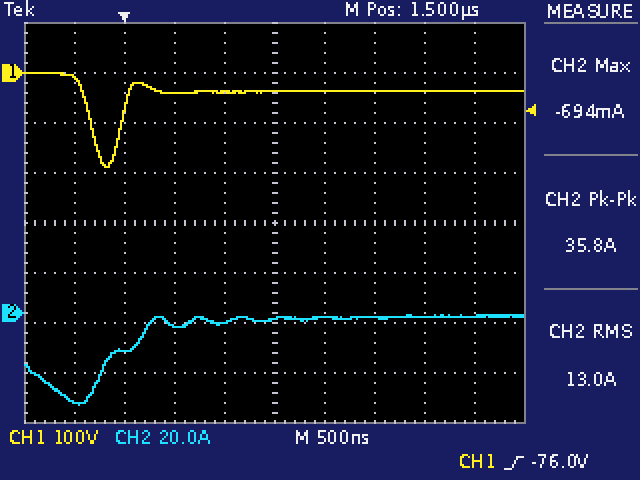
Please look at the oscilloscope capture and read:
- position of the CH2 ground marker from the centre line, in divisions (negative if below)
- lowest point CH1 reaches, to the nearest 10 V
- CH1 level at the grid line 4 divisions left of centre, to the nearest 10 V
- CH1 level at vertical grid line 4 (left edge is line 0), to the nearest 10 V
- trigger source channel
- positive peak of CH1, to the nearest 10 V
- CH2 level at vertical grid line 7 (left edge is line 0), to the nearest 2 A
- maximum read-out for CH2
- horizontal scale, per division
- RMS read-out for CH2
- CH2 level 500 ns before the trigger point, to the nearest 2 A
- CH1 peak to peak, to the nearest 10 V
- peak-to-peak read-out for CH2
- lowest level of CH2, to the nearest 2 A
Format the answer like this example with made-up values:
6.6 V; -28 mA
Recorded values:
-1.8 div; -190 V; -10 V; -40 V; CH1; 0 V; -2 A; -694 mA; 500 ns; 13.0 A; -36 A; 190 V; 35.8 A; -36 A
